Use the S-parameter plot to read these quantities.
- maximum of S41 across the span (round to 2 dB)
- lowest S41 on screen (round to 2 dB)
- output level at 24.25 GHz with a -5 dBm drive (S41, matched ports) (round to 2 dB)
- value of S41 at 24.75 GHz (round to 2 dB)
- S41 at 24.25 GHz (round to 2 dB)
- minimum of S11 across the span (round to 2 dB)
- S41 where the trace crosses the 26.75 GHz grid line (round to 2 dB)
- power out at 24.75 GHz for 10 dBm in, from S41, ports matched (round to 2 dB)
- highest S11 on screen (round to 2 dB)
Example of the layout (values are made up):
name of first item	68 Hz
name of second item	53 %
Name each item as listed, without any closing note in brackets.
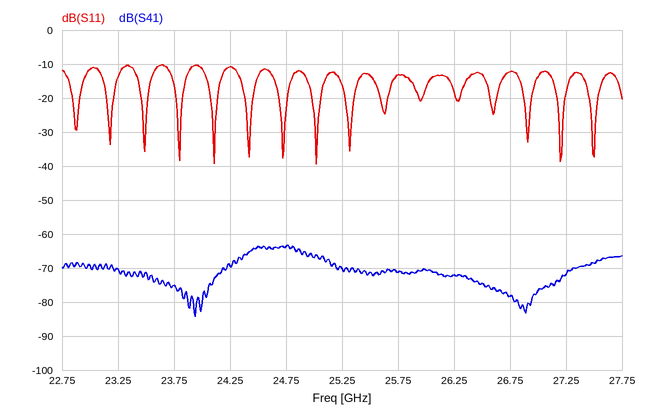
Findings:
maximum of S41 across the span	-64 dB
lowest S41 on screen	-84 dB
output level at 24.25 GHz with a -5 dBm drive (S41, matched ports)	-74 dBm
value of S41 at 24.75 GHz	-64 dB
S41 at 24.25 GHz	-70 dB
minimum of S11 across the span	-40 dB
S41 where the trace crosses the 26.75 GHz grid line	-78 dB
power out at 24.75 GHz for 10 dBm in, from S41, ports matched	-54 dBm
highest S11 on screen	-10 dB
